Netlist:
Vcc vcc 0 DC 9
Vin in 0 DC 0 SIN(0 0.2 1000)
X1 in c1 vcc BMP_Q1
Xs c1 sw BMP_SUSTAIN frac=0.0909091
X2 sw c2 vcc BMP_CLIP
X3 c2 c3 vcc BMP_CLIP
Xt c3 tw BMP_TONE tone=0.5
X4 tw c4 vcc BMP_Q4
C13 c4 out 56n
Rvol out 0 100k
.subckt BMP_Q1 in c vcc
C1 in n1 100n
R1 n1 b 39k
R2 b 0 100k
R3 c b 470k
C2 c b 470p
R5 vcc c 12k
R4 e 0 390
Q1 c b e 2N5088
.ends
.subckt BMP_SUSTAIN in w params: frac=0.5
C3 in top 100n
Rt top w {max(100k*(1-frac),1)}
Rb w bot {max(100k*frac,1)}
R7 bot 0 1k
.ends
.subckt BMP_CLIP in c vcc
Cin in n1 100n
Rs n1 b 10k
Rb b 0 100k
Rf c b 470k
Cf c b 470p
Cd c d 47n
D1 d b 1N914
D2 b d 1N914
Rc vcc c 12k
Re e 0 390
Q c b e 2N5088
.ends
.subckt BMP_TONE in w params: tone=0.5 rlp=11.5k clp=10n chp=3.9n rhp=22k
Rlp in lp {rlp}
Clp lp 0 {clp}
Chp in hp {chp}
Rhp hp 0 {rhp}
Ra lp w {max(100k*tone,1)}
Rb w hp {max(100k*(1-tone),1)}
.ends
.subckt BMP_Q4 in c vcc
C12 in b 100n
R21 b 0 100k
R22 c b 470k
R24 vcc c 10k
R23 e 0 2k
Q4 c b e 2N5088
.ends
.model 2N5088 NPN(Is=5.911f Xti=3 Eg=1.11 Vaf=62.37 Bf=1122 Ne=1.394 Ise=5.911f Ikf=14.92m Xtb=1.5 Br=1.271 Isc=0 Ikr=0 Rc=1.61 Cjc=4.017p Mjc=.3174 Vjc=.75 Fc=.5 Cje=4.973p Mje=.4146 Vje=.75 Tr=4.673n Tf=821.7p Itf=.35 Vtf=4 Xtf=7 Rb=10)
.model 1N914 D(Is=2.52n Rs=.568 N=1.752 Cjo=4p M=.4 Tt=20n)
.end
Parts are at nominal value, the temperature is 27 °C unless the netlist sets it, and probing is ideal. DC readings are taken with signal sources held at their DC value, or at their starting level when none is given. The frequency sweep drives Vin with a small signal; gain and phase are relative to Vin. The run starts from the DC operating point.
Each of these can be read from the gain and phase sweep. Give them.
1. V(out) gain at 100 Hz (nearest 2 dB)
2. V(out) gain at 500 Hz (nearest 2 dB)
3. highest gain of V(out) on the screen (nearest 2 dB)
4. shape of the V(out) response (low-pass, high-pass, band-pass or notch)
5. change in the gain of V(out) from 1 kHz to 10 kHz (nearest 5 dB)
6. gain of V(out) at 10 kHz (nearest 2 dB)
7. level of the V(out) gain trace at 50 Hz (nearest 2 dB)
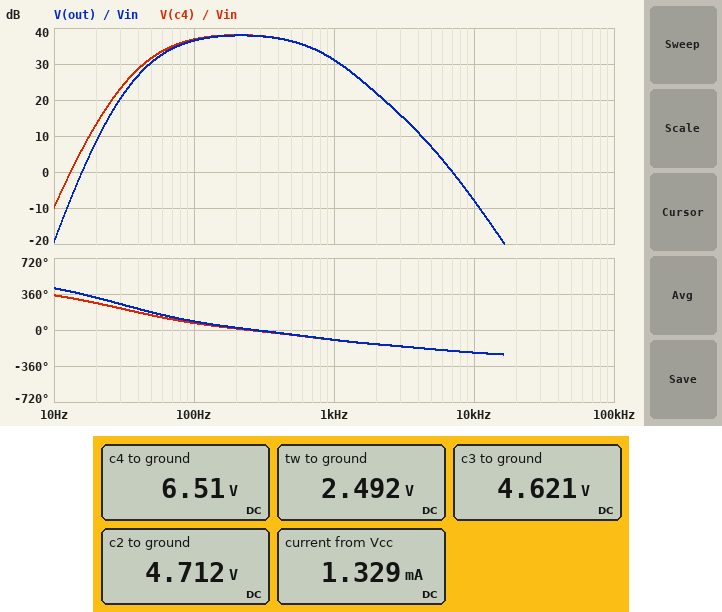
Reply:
36 dB
36 dB
38 dB
band-pass
-40 dB
-8 dB
30 dB
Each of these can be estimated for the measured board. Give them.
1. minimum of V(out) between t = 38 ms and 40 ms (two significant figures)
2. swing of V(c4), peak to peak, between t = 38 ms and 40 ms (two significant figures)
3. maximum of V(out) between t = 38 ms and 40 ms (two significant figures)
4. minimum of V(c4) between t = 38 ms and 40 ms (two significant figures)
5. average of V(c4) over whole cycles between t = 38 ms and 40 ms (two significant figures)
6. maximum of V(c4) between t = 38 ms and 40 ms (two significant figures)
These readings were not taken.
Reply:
-530 mV
1.1 V
520 mV
6.0 V
6.5 V
7.0 V
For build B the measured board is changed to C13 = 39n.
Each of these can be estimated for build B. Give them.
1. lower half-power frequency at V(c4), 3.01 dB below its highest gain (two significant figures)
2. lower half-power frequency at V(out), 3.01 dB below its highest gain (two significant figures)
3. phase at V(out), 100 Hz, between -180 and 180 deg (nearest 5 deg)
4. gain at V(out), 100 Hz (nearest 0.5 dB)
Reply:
70 Hz
80 Hz
90 deg
36.0 dB
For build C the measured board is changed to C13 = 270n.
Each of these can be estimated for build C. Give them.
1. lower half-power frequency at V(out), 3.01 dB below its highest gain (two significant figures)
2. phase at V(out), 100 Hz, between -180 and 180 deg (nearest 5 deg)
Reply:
72 Hz
75 deg
